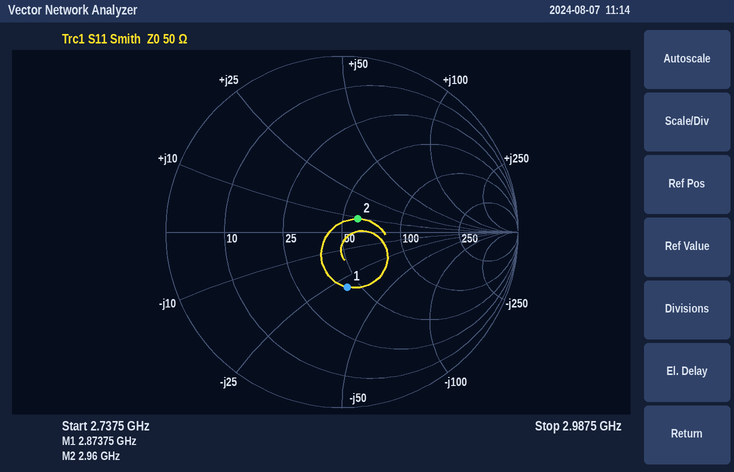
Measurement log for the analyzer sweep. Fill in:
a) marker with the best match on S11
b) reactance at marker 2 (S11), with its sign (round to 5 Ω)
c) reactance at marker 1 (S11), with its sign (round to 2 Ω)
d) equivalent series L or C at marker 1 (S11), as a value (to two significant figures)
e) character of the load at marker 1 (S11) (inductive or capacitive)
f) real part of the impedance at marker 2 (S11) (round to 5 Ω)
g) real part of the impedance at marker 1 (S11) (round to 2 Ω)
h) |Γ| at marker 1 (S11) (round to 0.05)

marker 2
+10 Ω
-30 Ω
1.8 pF
capacitive
60 Ω
44 Ω
0.30
